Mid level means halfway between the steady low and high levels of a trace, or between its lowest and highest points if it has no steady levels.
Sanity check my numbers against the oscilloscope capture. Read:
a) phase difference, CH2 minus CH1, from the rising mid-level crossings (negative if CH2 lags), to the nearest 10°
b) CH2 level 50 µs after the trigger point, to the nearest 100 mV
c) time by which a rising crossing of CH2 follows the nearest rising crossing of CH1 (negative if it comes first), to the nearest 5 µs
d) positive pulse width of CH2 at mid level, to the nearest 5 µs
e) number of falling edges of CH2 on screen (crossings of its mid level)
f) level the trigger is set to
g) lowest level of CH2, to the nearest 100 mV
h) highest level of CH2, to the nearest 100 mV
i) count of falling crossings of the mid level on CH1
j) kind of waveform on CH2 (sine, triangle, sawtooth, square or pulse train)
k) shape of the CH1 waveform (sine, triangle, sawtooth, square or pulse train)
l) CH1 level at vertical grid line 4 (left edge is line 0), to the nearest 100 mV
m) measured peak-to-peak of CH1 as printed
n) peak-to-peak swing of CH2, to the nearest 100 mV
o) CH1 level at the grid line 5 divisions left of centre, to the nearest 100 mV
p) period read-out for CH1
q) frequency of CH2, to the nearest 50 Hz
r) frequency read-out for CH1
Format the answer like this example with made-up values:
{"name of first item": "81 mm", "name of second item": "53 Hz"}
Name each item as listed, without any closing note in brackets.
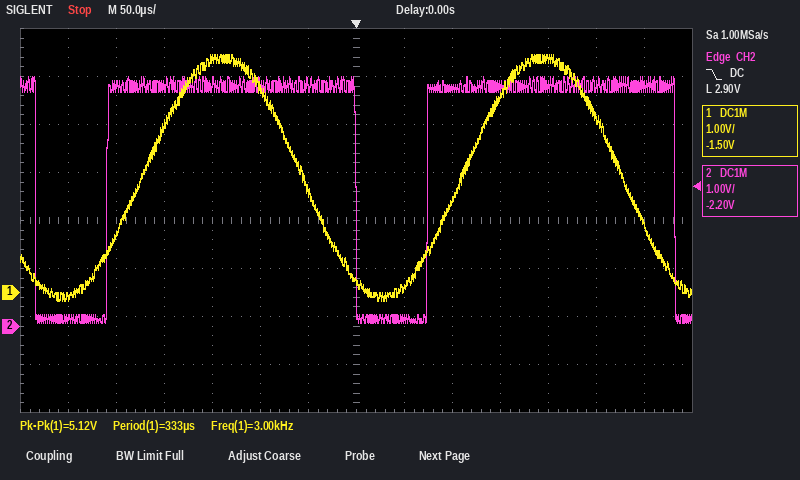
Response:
{"phase difference, CH2 minus CH1, from the rising mid-level crossings (negative if CH2 lags), to the nearest 10°": "+40°", "CH2 level 50 µs after the trigger point, to the nearest 100 mV": "200 mV", "time by which a rising crossing of CH2 follows the nearest rising crossing of CH1 (negative if it comes first), to the nearest 5 µs": "-35 µs", "positive pulse width of CH2 at mid level, to the nearest 5 µs": "260 µs", "number of falling edges of CH2 on screen": "3", "level the trigger is set to": "2.90 V", "lowest level of CH2, to the nearest 100 mV": "100 mV", "highest level of CH2, to the nearest 100 mV": "5.2 V", "count of falling crossings of the mid level on CH1": "2", "kind of waveform on CH2": "pulse train", "shape of the CH1 waveform": "sine", "CH1 level at vertical grid line 4 (left edge is line 0), to the nearest 100 mV": "4.9 V", "measured peak-to-peak of CH1 as printed": "5.12 V", "peak-to-peak swing of CH2, to the nearest 100 mV": "5.1 V", "CH1 level at the grid line 5 divisions left of centre, to the nearest 100 mV": "1.2 V", "period read-out for CH1": "333 µs", "frequency of CH2, to the nearest 50 Hz": "3.00 kHz", "frequency read-out for CH1": "3.00 kHz"}
